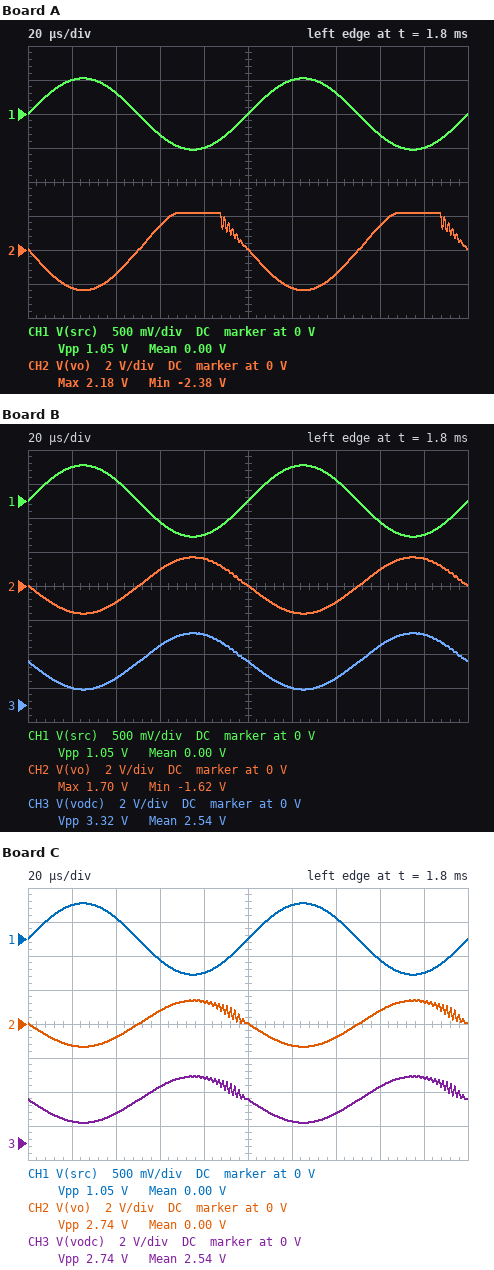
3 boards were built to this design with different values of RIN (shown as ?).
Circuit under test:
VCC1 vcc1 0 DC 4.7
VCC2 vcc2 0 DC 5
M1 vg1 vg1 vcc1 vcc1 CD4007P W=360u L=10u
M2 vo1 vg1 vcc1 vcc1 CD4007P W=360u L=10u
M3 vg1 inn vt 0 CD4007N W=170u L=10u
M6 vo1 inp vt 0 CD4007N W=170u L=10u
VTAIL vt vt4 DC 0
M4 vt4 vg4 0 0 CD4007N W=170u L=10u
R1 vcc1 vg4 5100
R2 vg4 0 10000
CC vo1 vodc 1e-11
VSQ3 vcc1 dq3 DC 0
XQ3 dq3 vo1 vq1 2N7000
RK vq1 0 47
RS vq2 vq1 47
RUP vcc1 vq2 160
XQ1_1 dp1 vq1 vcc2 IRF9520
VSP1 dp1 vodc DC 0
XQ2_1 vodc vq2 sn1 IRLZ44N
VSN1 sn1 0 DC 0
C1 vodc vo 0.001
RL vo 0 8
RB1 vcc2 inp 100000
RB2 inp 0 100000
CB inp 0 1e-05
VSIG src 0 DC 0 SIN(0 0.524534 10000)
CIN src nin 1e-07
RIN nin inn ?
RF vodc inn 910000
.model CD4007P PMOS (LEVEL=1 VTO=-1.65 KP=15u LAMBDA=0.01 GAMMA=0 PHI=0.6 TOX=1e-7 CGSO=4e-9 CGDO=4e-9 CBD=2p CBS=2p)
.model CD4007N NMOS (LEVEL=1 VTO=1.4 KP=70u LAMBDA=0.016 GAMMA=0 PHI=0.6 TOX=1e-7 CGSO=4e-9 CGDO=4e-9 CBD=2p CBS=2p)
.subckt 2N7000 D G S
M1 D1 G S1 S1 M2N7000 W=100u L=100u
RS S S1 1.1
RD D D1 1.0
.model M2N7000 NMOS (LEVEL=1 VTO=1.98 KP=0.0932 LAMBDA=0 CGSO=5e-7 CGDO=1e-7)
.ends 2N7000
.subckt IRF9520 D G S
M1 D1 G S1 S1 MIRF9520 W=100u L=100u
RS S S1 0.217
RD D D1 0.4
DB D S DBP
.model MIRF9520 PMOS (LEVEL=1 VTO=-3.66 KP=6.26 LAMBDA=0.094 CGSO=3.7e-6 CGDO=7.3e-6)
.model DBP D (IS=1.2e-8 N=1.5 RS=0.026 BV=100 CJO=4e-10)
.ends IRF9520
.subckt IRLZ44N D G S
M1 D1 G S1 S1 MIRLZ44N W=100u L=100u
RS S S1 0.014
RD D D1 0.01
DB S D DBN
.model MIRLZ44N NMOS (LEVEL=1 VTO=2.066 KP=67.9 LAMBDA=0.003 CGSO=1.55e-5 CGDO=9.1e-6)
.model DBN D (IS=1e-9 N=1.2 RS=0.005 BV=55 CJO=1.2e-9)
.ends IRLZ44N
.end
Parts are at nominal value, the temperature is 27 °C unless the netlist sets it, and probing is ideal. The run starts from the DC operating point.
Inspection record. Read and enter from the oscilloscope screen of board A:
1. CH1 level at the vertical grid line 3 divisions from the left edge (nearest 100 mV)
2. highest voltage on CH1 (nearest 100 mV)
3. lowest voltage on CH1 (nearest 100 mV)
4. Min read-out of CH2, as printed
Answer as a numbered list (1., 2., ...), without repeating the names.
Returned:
1. -300 mV
2. 500 mV
3. -500 mV
4. -2.38 V
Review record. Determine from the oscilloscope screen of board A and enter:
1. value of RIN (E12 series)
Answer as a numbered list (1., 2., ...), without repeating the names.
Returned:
1. 180 kΩ
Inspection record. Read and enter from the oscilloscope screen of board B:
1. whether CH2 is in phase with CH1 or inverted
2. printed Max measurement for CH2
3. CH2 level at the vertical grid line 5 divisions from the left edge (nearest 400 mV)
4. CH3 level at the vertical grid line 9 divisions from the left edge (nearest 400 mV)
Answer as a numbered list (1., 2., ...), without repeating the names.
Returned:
1. inverted
2. 1.70 V
3. 0 V
4. 4.0 V
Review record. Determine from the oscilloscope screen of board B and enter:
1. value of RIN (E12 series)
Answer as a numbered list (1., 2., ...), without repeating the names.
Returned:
1. 270 kΩ
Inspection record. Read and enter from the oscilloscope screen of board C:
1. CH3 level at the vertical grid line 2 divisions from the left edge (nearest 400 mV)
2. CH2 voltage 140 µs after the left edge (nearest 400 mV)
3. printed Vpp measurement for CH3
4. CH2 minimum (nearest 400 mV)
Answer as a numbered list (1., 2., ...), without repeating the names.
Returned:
1. 1.6 V
2. -800 mV
3. 2.74 V
4. -1.2 V
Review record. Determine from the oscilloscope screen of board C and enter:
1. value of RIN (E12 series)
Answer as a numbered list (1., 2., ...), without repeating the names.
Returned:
1. 330 kΩ
